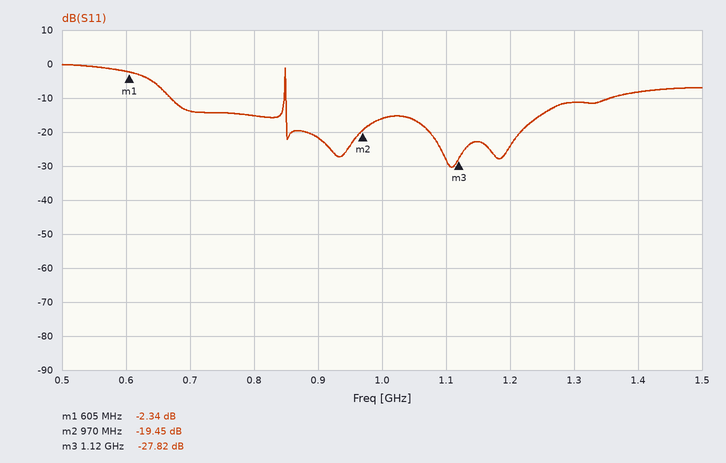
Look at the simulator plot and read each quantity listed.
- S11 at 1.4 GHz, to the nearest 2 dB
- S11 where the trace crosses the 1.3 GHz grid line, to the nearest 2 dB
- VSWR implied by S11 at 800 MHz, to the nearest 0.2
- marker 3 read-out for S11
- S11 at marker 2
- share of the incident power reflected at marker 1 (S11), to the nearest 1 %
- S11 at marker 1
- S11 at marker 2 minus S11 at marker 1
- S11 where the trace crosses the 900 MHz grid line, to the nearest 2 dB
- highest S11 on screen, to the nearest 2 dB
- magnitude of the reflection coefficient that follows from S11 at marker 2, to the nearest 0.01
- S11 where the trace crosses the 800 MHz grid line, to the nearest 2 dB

-8 dB
-12 dB
1.4
-27.82 dB
-19.45 dB
58 %
-2.34 dB
-17.11 dB
-22 dB
0 dB
0.11
-16 dB
